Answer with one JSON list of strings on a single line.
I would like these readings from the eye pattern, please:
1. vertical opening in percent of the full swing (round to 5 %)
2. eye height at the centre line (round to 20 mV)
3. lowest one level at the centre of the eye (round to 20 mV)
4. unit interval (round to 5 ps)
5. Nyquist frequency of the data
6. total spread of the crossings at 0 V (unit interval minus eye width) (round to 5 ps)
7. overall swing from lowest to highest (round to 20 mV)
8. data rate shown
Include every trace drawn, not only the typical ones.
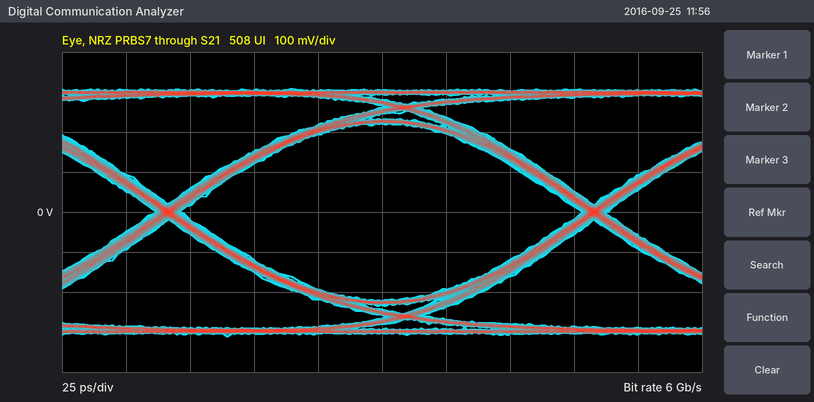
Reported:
["70 %", "440 mV", "220 mV", "165 ps", "3 GHz", "10 ps", "620 mV", "6 Gb/s"]
